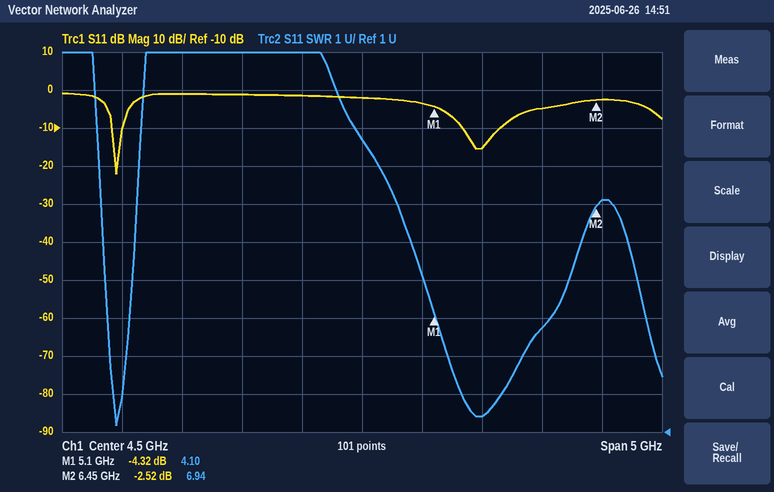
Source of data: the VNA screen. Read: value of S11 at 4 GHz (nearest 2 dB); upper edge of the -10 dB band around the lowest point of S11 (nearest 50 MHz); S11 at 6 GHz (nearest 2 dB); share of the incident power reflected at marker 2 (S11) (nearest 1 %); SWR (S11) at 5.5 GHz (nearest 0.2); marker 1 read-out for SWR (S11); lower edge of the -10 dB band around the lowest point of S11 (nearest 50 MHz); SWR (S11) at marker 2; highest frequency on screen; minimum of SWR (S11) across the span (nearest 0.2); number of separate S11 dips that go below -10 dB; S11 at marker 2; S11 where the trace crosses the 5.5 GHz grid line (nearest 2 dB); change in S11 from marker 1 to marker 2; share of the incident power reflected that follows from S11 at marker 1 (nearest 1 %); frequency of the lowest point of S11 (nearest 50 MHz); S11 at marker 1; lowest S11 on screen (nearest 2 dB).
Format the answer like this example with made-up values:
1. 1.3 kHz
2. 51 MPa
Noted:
1. -2 dB
2. 2.50 GHz
3. -4 dB
4. 56 %
5. 1.4
6. 4.10
7. 2.40 GHz
8. 6.94
9. 7 GHz
10. 1.2
11. 2
12. -2.52 dB
13. -16 dB
14. 1.80 dB
15. 37 %
16. 2.45 GHz
17. -4.32 dB
18. -22 dB
